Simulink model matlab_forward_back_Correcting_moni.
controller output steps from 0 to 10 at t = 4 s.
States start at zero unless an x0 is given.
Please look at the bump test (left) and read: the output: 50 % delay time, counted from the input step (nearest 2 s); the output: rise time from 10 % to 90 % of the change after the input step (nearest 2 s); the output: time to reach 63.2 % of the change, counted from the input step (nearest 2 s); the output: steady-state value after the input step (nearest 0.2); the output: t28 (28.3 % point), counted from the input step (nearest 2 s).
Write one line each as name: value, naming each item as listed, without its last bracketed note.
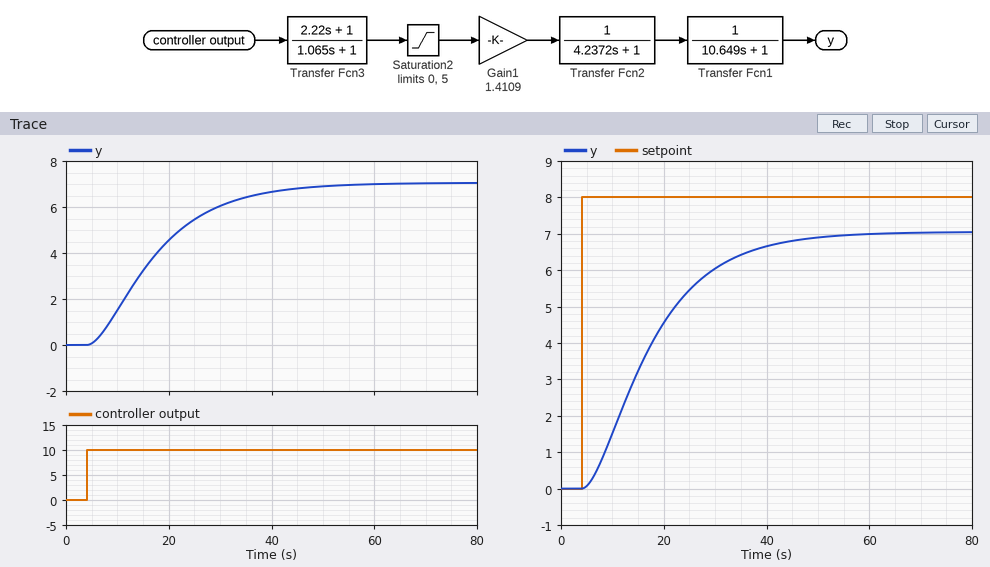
the output: 50 % delay time, counted from the input step: 12 s
the output: rise time from 10 % to 90 % of the change after the input step: 26 s
the output: time to reach 63.2 % of the change, counted from the input step: 16 s
the output: steady-state value after the input step: 7.0
the output: t28 (28.3 % point), counted from the input step: 8 s
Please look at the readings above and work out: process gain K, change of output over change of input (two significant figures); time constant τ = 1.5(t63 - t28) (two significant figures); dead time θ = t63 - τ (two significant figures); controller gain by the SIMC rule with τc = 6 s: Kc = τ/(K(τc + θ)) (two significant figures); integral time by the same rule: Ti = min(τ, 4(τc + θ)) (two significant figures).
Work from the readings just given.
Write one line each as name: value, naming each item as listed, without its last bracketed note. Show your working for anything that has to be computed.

process gain K, change of output over change of input: (7 - 0) / 10 = 0.70
time constant τ = 1.5(t63 - t28): 1.5 × (16 - 8) = 12 s
dead time θ = t63 - τ: 16 - 12 = 4.0 s
controller gain by the SIMC rule with τc = 6 s: Kc = τ/(K(τc + θ)): 12 / (0.7 × (6 + 4)) = 1.7
integral time by the same rule: Ti = min(τ, 4(τc + θ)): min(12, 4 × (6 + 4)) = 12 s
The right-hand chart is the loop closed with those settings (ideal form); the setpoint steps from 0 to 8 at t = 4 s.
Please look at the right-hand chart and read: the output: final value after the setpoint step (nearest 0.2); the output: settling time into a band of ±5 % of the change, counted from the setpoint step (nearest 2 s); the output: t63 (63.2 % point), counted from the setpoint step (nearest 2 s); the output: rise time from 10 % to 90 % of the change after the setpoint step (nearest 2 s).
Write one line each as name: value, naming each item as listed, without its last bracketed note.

the output: final value after the setpoint step: 7.0
the output: settling time into a band of ±5 % of the change, counted from the setpoint step: 38 s
the output: t63 (63.2 % point), counted from the setpoint step: 16 s
the output: rise time from 10 % to 90 % of the change after the setpoint step: 26 s
